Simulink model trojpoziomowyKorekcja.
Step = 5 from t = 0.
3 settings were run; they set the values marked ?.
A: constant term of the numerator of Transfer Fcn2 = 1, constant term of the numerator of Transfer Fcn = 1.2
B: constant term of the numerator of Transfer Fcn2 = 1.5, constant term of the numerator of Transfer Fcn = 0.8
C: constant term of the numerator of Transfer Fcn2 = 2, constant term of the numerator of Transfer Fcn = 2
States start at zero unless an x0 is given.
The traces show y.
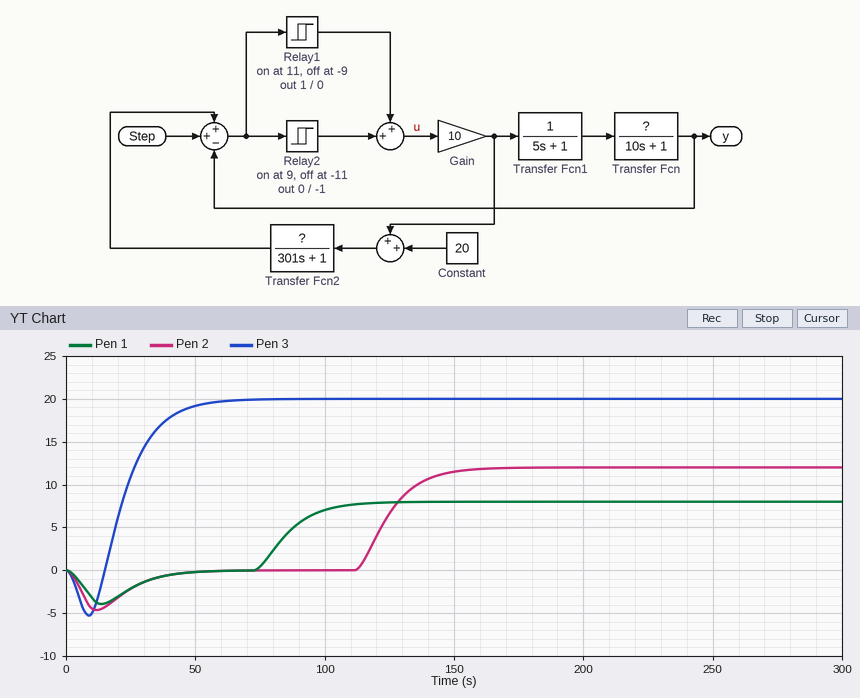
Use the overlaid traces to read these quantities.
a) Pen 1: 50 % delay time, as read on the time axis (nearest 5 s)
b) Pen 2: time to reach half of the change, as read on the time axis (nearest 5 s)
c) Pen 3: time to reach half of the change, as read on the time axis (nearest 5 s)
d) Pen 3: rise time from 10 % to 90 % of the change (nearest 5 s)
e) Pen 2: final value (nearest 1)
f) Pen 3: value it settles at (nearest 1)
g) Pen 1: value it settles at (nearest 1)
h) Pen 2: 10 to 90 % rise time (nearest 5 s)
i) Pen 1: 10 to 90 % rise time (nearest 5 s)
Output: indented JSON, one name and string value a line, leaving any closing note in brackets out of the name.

{
  "Pen 1: 50 % delay time, as read on the time axis": "85 s",
  "Pen 2: time to reach half of the change, as read on the time axis": "125 s",
  "Pen 3: time to reach half of the change, as read on the time axis": "25 s",
  "Pen 3: rise time from 10 % to 90 % of the change": "25 s",
  "Pen 2: final value": "12",
  "Pen 3: value it settles at": "20",
  "Pen 1: value it settles at": "8",
  "Pen 2: 10 to 90 % rise time": "25 s",
  "Pen 1: 10 to 90 % rise time": "25 s"
}
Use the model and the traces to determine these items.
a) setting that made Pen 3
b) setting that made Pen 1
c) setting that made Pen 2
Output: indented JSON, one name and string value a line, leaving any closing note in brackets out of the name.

{
  "setting that made Pen 3": "C",
  "setting that made Pen 1": "B",
  "setting that made Pen 2": "A"
}
